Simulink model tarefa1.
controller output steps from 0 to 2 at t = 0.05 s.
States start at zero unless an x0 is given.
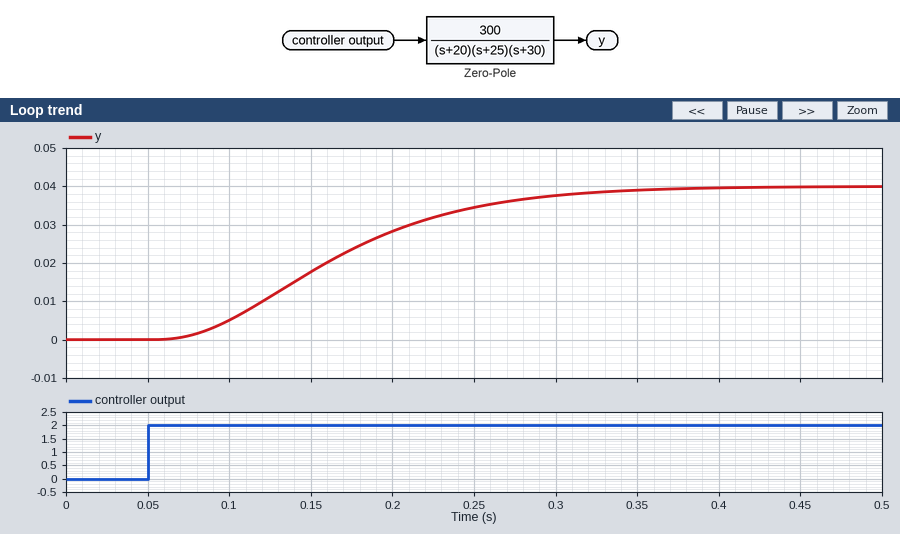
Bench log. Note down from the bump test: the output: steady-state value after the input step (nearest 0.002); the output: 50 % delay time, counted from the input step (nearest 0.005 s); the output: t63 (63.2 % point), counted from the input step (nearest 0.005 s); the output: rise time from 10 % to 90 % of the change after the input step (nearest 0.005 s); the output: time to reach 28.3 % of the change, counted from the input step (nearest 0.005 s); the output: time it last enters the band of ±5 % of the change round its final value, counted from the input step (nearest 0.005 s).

0.040
0.110 s
0.135 s
0.175 s
0.075 s
0.260 s
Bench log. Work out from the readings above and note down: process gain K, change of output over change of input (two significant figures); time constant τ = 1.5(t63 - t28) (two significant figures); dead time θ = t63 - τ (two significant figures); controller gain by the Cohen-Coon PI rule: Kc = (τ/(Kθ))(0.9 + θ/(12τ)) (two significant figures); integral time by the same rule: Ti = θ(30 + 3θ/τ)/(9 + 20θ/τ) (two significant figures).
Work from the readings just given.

0.020
0.090 s
0.045 s
94
0.075 s
